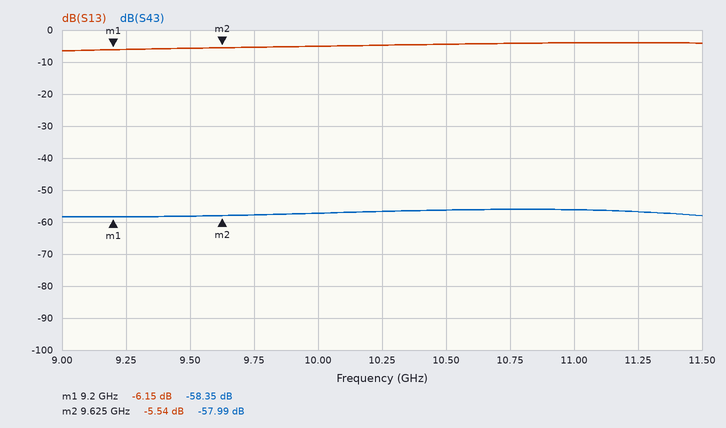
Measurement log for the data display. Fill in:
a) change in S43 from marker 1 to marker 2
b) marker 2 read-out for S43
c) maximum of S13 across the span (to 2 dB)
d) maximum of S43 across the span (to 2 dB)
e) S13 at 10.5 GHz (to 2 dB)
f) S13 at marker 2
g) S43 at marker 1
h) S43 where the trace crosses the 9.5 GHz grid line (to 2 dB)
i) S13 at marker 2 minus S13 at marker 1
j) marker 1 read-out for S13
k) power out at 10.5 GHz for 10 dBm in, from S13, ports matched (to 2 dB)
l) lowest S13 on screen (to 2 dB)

0.36 dB
-57.99 dB
-4 dB
-56 dB
-4 dB
-5.54 dB
-58.35 dB
-58 dB
0.61 dB
-6.15 dB
6 dBm
-6 dB
